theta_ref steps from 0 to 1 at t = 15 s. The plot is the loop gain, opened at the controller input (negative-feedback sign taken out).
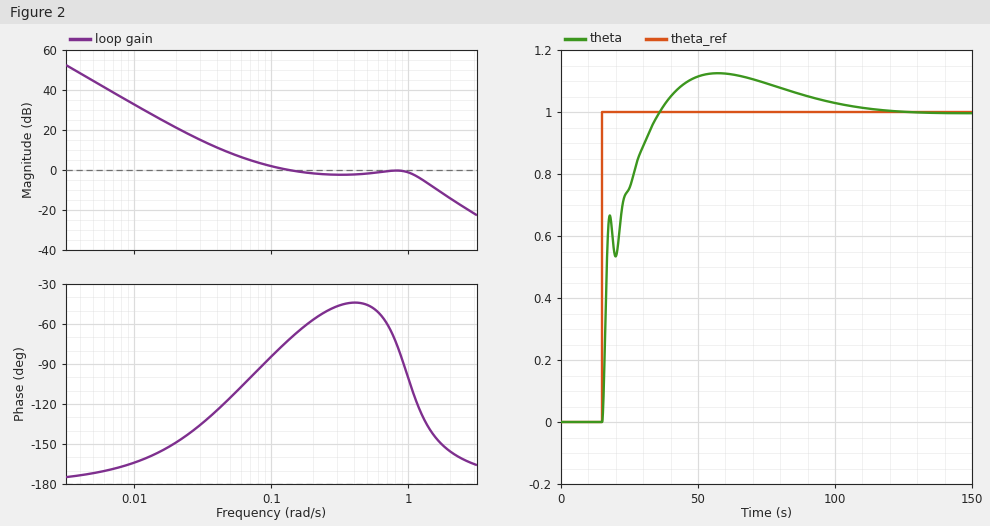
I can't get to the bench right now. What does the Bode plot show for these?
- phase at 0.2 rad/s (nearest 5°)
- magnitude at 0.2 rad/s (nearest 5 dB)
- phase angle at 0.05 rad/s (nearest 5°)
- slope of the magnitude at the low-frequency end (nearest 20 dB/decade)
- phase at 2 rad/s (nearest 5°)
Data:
-55°
0 dB
-115°
-40 dB/decade
-155°
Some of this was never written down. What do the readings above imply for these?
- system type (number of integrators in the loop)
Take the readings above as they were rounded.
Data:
2
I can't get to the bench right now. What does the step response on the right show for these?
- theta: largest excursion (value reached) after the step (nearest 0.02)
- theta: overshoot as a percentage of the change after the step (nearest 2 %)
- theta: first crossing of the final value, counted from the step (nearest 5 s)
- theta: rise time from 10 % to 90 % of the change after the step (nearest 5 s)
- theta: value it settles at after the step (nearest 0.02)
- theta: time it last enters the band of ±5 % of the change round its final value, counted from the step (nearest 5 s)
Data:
1.12
12 %
20 s
15 s
1.00
75 s
